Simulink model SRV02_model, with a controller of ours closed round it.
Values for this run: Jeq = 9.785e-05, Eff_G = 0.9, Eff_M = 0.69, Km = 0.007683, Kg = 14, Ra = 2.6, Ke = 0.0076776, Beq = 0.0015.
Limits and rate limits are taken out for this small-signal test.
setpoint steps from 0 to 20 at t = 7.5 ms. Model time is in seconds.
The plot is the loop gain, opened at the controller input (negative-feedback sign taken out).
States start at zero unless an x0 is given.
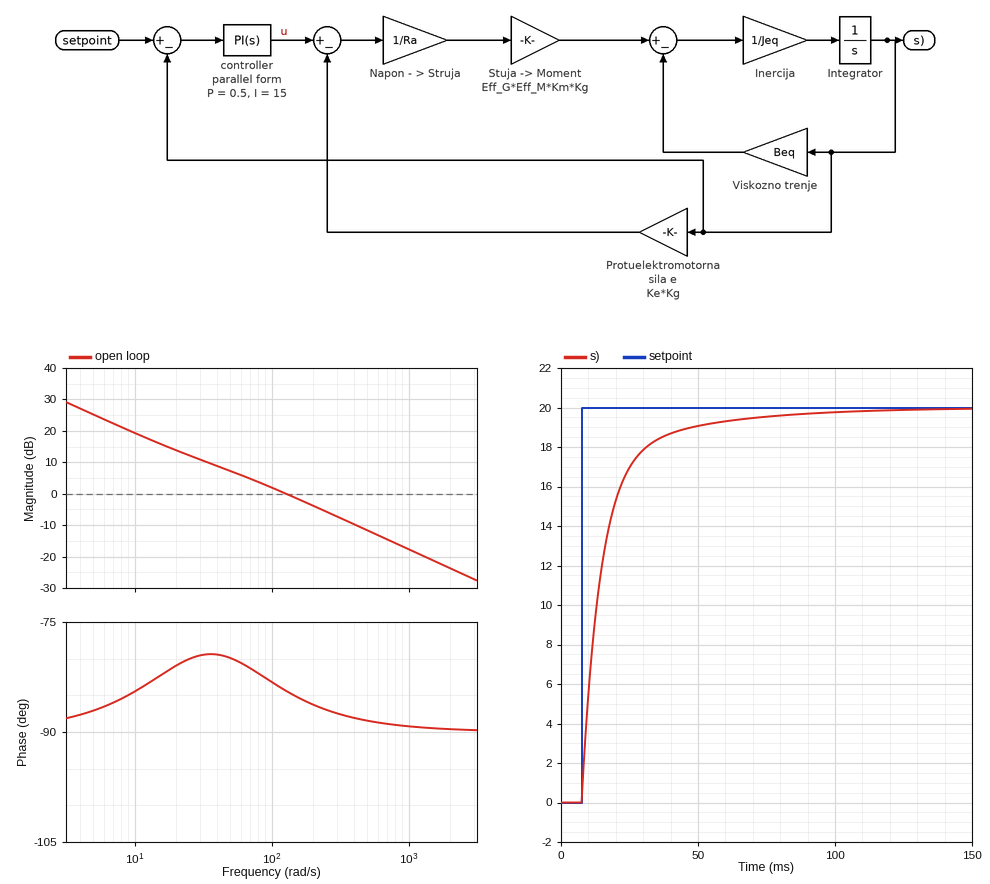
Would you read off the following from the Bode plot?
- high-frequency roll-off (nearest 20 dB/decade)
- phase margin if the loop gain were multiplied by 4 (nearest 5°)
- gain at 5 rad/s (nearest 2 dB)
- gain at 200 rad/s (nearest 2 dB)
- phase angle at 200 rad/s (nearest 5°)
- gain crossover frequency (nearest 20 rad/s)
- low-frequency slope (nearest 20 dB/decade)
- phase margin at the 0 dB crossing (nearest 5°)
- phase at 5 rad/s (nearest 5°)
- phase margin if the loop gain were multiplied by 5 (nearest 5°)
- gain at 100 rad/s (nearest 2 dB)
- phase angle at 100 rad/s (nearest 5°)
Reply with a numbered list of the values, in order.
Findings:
1. -20 dB/decade
2. 90°
3. 26 dB
4. -4 dB
5. -85°
6. 120 rad/s
7. -20 dB/decade
8. 95°
9. -85°
10. 90°
11. 2 dB
12. -85°
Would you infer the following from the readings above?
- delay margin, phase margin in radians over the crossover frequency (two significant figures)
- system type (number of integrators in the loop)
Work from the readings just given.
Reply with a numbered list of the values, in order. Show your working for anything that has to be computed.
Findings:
1. 95 × π / 180 / 120 = 0.014 s
2. 1
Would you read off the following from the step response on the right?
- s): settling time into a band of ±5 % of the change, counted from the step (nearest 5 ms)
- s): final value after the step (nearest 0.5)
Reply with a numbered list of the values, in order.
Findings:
1. 40 ms
2. 20.0
